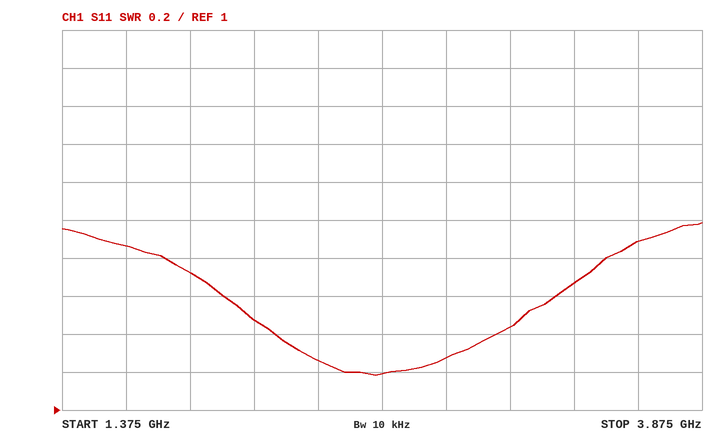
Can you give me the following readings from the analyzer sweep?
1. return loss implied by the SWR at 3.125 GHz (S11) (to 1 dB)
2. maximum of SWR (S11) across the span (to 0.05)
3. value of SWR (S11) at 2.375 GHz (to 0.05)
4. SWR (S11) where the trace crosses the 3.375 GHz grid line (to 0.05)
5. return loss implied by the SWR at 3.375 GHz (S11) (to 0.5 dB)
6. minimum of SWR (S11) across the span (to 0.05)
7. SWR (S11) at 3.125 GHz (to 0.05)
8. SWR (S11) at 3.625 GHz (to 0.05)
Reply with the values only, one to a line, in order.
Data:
15 dB
2.00
1.25
1.65
12.0 dB
1.20
1.45
1.90
